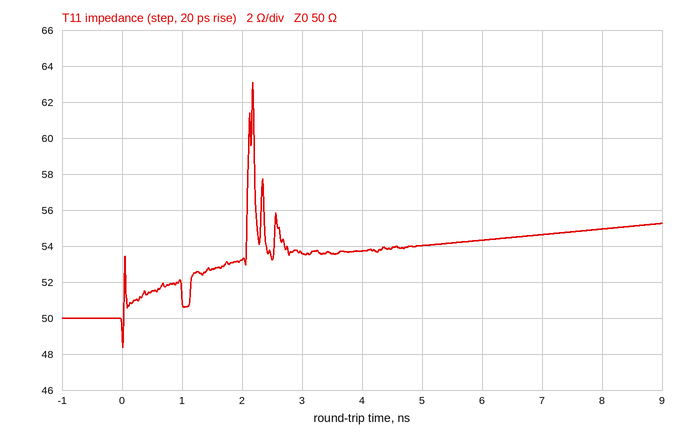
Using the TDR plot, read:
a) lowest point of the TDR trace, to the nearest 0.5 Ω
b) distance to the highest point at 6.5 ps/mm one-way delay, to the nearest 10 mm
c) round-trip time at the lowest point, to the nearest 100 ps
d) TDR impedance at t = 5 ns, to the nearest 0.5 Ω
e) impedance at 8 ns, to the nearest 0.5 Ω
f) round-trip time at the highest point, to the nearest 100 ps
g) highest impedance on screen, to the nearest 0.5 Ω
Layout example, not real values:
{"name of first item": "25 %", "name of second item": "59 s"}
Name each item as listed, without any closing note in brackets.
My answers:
{"lowest point of the TDR trace, to the nearest 0.5 Ω": "48.5 Ω", "distance to the highest point at 6.5 ps/mm one-way delay, to the nearest 10 mm": "170 mm", "round-trip time at the lowest point, to the nearest 100 ps": "0.0 ns", "TDR impedance at t = 5 ns, to the nearest 0.5 Ω": "54.0 Ω", "impedance at 8 ns, to the nearest 0.5 Ω": "55.0 Ω", "round-trip time at the highest point, to the nearest 100 ps": "2.2 ns", "highest impedance on screen, to the nearest 0.5 Ω": "63.0 Ω"}
